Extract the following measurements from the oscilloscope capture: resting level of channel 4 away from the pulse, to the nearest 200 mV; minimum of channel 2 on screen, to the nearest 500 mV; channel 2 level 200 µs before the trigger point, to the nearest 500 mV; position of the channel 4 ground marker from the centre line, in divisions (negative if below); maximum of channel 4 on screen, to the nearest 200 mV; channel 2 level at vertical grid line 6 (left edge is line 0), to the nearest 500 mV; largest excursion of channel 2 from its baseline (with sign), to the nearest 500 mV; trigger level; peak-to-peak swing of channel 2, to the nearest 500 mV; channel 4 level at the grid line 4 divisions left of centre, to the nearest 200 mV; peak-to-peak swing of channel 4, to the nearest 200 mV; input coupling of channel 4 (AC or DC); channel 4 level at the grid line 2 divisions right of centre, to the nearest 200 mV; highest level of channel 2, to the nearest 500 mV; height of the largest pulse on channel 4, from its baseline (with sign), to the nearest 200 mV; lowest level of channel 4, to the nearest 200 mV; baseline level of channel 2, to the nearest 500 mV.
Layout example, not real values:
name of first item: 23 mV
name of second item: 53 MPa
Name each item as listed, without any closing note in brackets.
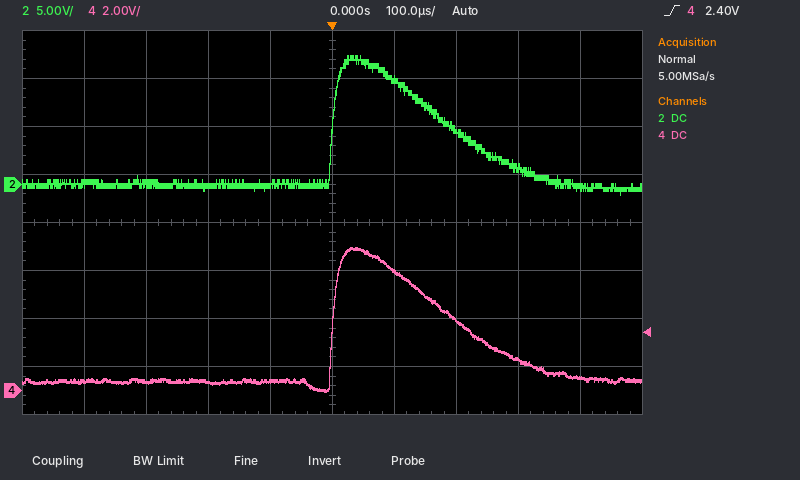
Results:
resting level of channel 4 away from the pulse, to the nearest 200 mV: 400 mV
minimum of channel 2 on screen, to the nearest 500 mV: -1.0 V
channel 2 level 200 µs before the trigger point, to the nearest 500 mV: 0.0 V
position of the channel 4 ground marker from the centre line, in divisions: -3.5 div
maximum of channel 4 on screen, to the nearest 200 mV: 6.0 V
channel 2 level at vertical grid line 6 (left edge is line 0), to the nearest 500 mV: 11.0 V
largest excursion of channel 2 from its baseline (with sign), to the nearest 500 mV: +13.5 V
trigger level: 2.40 V
peak-to-peak swing of channel 2, to the nearest 500 mV: 14.5 V
channel 4 level at the grid line 4 divisions left of centre, to the nearest 200 mV: 400 mV
peak-to-peak swing of channel 4, to the nearest 200 mV: 6.0 V
input coupling of channel 4: DC
channel 4 level at the grid line 2 divisions right of centre, to the nearest 200 mV: 3.0 V
highest level of channel 2, to the nearest 500 mV: 13.5 V
height of the largest pulse on channel 4, from its baseline (with sign), to the nearest 200 mV: +5.6 V
lowest level of channel 4, to the nearest 200 mV: 0.0 V
baseline level of channel 2, to the nearest 500 mV: 0.0 V
